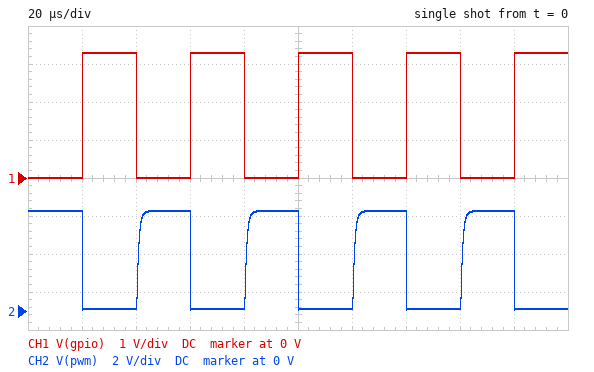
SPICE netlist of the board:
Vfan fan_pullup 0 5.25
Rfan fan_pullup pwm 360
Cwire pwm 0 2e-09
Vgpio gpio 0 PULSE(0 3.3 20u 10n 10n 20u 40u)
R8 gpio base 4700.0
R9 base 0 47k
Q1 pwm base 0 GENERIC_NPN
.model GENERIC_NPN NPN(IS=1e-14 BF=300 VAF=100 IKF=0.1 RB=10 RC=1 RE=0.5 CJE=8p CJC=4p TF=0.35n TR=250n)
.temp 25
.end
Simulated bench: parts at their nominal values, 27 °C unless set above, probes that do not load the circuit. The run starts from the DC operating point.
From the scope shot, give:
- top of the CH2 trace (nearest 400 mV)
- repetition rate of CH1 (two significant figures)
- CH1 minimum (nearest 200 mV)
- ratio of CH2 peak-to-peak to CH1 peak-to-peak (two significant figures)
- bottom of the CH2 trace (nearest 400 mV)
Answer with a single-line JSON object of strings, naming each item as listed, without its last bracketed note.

{"top of the CH2 trace": "5.2 V", "repetition rate of CH1": "25 kHz", "CH1 minimum": "0 V", "ratio of CH2 peak-to-peak to CH1 peak-to-peak": "1.6", "bottom of the CH2 trace": "0 V"}
